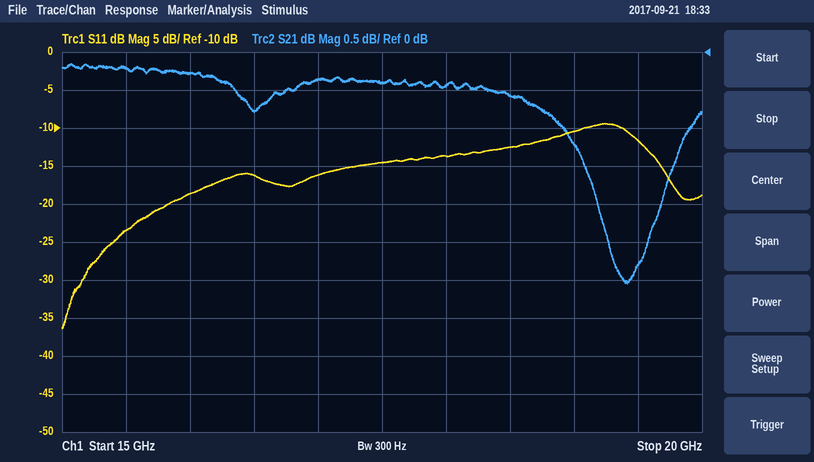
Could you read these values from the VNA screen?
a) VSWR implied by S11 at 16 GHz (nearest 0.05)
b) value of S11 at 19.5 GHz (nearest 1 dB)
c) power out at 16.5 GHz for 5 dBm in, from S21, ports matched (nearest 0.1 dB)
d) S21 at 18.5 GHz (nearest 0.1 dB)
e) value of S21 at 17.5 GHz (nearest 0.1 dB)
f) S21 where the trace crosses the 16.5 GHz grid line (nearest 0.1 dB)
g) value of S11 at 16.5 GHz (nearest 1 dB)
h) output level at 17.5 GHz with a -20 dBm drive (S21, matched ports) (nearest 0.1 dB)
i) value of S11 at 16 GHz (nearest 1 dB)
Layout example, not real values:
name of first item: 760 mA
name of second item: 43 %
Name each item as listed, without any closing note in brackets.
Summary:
VSWR implied by S11 at 16 GHz: 1.25
value of S11 at 19.5 GHz: -12 dB
power out at 16.5 GHz for 5 dBm in, from S21, ports matched: 4.2 dBm
S21 at 18.5 GHz: -0.6 dB
value of S21 at 17.5 GHz: -0.4 dB
S21 where the trace crosses the 16.5 GHz grid line: -0.8 dB
value of S11 at 16.5 GHz: -16 dB
output level at 17.5 GHz with a -20 dBm drive (S21, matched ports): -20.4 dBm
value of S11 at 16 GHz: -19 dB
